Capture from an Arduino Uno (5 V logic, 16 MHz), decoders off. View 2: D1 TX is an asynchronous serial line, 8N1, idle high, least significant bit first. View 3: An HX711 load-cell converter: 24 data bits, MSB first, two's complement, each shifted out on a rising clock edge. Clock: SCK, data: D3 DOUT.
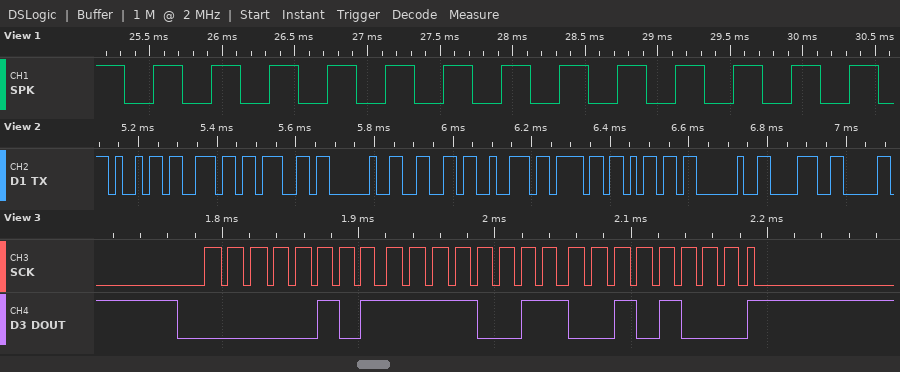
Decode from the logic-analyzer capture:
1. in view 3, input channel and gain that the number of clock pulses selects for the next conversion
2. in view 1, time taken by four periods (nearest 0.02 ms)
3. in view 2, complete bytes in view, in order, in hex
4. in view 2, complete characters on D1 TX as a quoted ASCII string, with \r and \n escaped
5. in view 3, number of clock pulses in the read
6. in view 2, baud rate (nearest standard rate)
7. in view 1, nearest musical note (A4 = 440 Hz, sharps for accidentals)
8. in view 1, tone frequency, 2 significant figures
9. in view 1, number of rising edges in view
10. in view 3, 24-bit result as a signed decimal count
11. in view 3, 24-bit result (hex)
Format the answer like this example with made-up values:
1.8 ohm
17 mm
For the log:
channel A, gain 128
1.60 ms
69 6E 67 20 66 72 6F 6D 20 38
"ing from 8"
25
57600 baud
D#7
2.5 kHz
13
389928
0x05F328
